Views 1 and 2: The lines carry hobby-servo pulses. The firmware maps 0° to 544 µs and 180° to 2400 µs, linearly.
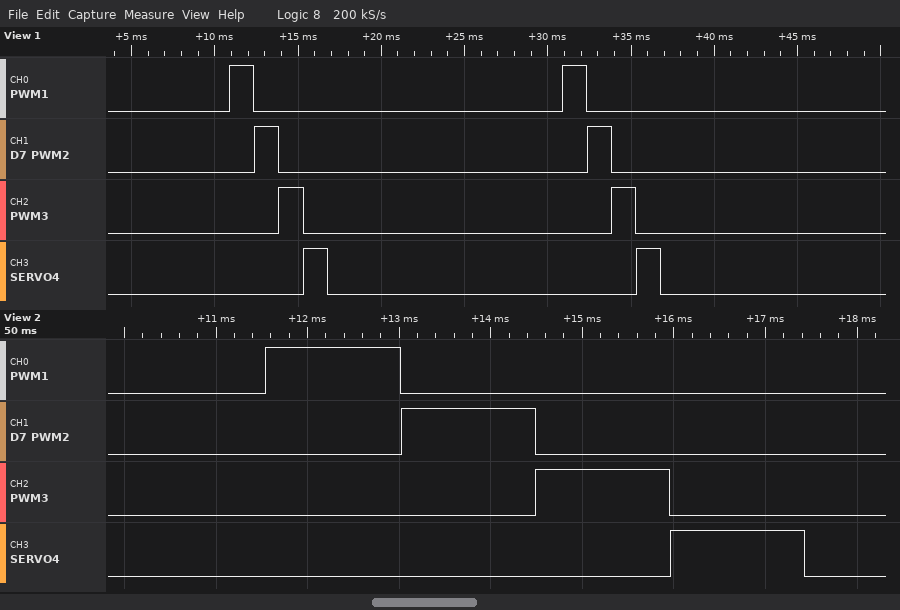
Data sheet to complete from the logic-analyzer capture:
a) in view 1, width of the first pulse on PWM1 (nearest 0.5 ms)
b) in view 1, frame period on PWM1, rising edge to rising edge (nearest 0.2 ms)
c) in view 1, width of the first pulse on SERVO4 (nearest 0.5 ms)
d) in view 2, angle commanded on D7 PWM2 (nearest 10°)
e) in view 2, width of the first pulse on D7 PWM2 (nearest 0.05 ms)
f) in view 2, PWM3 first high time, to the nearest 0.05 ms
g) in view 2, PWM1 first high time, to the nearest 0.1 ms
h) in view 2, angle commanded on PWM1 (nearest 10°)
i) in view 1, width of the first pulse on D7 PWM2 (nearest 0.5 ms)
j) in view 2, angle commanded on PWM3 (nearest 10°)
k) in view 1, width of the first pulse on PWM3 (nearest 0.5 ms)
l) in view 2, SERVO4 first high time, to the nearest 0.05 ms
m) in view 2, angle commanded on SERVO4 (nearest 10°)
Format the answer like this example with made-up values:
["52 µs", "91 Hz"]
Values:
["1.5 ms", "20.0 ms", "1.5 ms", "90°", "1.45 ms", "1.45 ms", "1.5 ms", "90°", "1.5 ms", "90°", "1.5 ms", "1.45 ms", "90°"]
